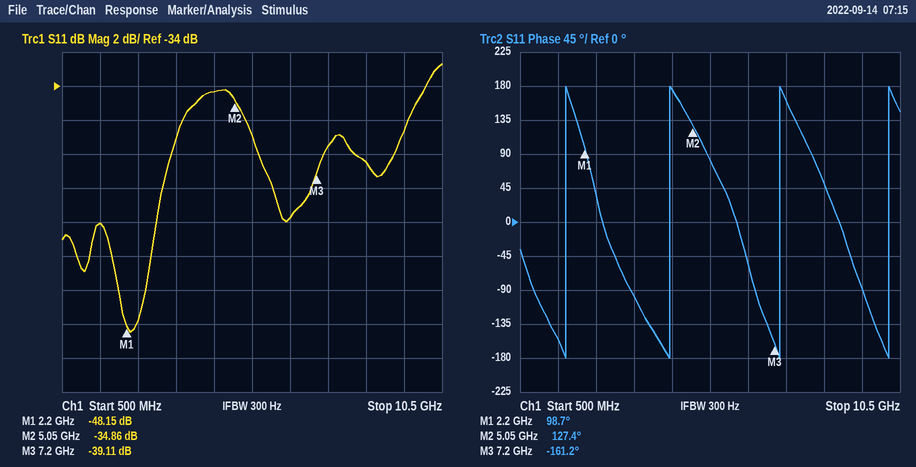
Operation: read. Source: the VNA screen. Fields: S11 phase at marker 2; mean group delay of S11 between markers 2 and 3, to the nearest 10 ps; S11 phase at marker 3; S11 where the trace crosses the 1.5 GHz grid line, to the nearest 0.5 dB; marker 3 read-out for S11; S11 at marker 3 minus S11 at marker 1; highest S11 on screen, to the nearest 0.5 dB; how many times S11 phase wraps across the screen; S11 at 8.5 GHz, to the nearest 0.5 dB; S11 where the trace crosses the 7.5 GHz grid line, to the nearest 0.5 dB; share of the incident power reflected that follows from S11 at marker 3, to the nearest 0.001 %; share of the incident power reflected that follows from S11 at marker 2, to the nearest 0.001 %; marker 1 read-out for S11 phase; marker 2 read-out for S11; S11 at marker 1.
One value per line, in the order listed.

127.4°
370 ps
-161.2°
-42.0 dB
-39.11 dB
9.04 dB
-32.5 dB
4
-38.5 dB
-37.5 dB
0.012 %
0.033 %
98.7°
-34.86 dB
-48.15 dB
